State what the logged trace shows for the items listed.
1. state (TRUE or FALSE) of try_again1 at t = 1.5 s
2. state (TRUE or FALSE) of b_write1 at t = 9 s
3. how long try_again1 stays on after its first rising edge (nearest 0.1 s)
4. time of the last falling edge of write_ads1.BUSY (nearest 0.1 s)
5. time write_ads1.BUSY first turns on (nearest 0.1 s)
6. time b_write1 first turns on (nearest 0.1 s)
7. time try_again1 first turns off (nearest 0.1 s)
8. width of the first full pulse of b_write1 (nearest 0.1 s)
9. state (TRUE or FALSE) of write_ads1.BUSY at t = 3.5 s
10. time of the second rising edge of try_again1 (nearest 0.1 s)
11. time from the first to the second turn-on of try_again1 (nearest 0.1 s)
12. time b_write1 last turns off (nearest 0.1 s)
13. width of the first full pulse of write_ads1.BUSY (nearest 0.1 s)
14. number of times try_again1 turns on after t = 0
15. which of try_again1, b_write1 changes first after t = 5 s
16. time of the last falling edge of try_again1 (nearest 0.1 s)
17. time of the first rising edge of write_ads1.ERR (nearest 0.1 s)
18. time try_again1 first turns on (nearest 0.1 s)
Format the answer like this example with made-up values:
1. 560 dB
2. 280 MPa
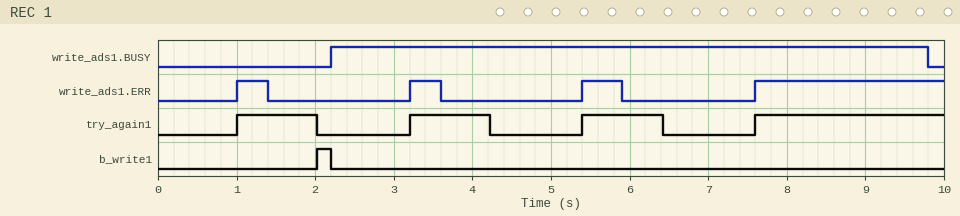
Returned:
1. TRUE
2. FALSE
3. 1.0 s
4. 9.8 s
5. 2.2 s
6. 2.0 s
7. 2.0 s
8. 0.2 s
9. TRUE
10. 3.2 s
11. 2.2 s
12. 2.2 s
13. 7.6 s
14. 4
15. try_again1
16. 6.4 s
17. 1.0 s
18. 1.0 s
